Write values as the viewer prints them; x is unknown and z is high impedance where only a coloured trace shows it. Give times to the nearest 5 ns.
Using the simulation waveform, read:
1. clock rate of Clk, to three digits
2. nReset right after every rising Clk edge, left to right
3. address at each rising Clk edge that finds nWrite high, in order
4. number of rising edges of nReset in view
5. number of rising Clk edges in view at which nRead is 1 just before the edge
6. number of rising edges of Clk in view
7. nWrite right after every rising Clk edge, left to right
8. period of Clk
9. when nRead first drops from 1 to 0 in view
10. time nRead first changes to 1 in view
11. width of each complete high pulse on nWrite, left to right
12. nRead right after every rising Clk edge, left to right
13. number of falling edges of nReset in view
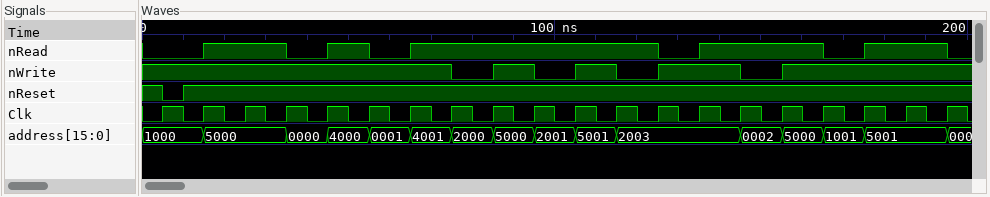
100 MHz
0 1 1 1 1 1 1 1 1 1 1 1 1 1 1 1 1 1 1 1
1000, 1000, 5000, 5000, 0000, 4000, 0001, 4001, 5000, 5001, 2003, 2003, 5000, 1001, 5001, 5001
1
14
20
1 1 1 1 1 1 1 0 1 0 1 0 1 1 0 1 1 1 1 1
10 ns
35 ns
15 ns
10 ns, 10 ns, 20 ns
0 1 1 0 1 0 1 1 1 1 1 1 0 1 1 1 0 1 1 0
1
